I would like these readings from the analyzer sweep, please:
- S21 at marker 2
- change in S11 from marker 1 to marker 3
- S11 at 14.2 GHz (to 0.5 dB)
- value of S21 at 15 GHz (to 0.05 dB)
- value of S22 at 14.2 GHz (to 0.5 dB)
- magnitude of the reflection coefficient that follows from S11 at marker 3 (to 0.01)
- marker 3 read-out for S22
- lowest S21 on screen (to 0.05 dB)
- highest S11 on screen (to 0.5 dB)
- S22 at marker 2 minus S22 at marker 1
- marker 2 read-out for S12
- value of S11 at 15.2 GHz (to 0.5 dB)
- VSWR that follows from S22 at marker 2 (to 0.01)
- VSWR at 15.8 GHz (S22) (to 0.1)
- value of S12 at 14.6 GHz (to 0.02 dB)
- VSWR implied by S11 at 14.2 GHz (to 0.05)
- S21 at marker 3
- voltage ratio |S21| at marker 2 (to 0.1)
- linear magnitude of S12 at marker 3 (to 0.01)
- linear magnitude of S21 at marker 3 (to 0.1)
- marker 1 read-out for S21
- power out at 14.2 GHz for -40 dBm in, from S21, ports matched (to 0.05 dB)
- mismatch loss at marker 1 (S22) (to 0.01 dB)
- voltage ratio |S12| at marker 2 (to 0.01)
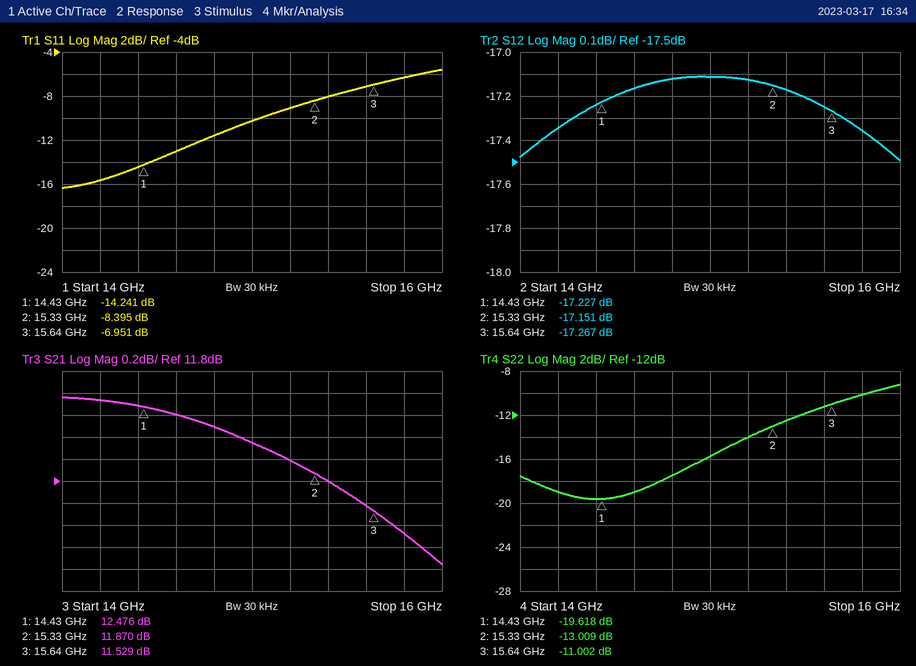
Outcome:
11.870 dB
7.290 dB
-15.5 dB
12.15 dB
-19.0 dB
0.45
-11.002 dB
11.05 dB
-5.5 dB
6.609 dB
-17.151 dB
-9.0 dB
1.58
1.9
-17.16 dB
1.40
11.529 dB
3.9
0.14
3.8
12.476 dB
-27.45 dBm
0.05 dB
0.14
